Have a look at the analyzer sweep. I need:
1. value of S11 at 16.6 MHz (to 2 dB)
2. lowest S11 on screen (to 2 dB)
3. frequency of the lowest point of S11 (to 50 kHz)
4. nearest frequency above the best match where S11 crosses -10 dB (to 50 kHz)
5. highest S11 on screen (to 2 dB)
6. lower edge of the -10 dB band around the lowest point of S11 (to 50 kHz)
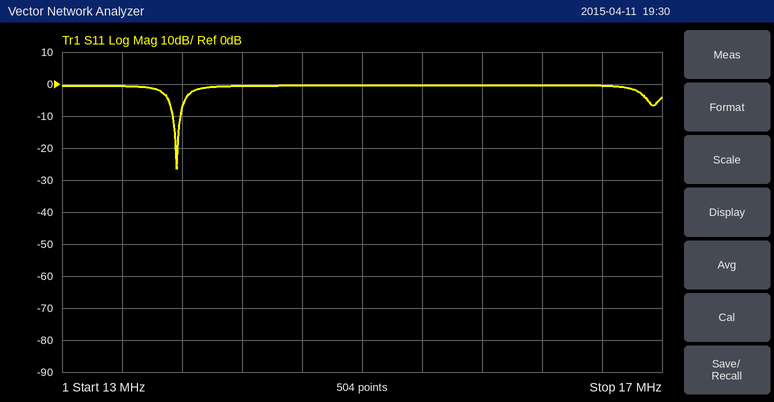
0 dB
-26 dB
13.75 MHz
13.80 MHz
0 dB
13.75 MHz
